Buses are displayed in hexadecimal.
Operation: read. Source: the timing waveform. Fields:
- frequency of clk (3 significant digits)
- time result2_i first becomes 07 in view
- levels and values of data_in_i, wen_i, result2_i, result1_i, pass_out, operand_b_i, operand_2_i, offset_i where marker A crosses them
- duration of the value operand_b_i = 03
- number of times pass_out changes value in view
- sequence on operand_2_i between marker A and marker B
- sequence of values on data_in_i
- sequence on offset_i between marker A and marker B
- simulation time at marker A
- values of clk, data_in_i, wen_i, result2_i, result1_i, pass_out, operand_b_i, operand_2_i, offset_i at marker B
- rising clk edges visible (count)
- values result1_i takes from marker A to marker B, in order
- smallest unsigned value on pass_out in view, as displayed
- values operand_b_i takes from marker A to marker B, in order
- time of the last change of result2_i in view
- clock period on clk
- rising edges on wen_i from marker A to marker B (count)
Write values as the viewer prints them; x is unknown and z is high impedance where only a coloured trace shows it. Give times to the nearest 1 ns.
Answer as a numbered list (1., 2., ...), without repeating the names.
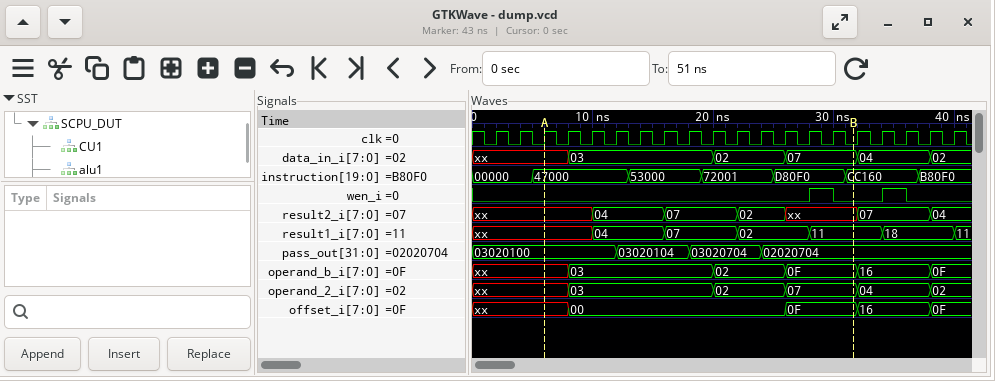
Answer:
1. 500 MHz
2. 16 ns
3. data_in_i=xx, wen_i=0, result2_i=xx, result1_i=xx, pass_out=03020100, operand_b_i=xx, operand_2_i=xx, offset_i=xx
4. 12 ns
5. 3
6. xx, 03, 02, 07
7. xx, 03, 02, 07, 04, 02
8. xx, 00, 0F
9. 6 ns
10. clk=0, data_in_i=07, wen_i=0, result2_i=xx, result1_i=11, pass_out=02020704, operand_b_i=0F, operand_2_i=07, offset_i=0F
11. 20
12. xx, 04, 07, 02, 11
13. 02020704
14. xx, 03, 02, 0F
15. 38 ns
16. 2 ns
17. 1
